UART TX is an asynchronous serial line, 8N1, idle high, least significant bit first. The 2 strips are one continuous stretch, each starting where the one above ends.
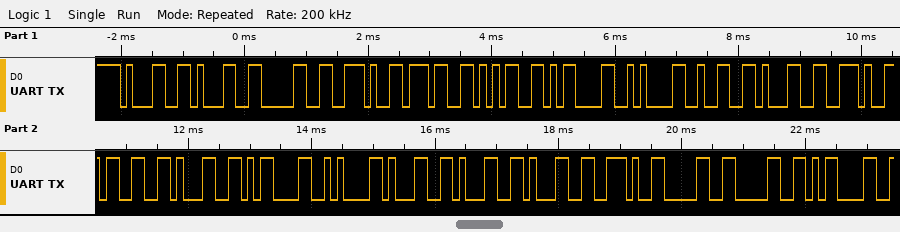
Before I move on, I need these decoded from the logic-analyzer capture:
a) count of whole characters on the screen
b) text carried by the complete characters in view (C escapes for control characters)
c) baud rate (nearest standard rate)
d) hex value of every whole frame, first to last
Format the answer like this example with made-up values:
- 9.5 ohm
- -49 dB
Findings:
- 22
- "110.75\r\n21.31\r\n111.00\r"
- 9600 baud
- 0x31 0x31 0x30 0x2E 0x37 0x35 0x0D 0x0A 0x32 0x31 0x2E 0x33 0x31 0x0D 0x0A 0x31 0x31 0x31 0x2E 0x30 0x30 0x0D
